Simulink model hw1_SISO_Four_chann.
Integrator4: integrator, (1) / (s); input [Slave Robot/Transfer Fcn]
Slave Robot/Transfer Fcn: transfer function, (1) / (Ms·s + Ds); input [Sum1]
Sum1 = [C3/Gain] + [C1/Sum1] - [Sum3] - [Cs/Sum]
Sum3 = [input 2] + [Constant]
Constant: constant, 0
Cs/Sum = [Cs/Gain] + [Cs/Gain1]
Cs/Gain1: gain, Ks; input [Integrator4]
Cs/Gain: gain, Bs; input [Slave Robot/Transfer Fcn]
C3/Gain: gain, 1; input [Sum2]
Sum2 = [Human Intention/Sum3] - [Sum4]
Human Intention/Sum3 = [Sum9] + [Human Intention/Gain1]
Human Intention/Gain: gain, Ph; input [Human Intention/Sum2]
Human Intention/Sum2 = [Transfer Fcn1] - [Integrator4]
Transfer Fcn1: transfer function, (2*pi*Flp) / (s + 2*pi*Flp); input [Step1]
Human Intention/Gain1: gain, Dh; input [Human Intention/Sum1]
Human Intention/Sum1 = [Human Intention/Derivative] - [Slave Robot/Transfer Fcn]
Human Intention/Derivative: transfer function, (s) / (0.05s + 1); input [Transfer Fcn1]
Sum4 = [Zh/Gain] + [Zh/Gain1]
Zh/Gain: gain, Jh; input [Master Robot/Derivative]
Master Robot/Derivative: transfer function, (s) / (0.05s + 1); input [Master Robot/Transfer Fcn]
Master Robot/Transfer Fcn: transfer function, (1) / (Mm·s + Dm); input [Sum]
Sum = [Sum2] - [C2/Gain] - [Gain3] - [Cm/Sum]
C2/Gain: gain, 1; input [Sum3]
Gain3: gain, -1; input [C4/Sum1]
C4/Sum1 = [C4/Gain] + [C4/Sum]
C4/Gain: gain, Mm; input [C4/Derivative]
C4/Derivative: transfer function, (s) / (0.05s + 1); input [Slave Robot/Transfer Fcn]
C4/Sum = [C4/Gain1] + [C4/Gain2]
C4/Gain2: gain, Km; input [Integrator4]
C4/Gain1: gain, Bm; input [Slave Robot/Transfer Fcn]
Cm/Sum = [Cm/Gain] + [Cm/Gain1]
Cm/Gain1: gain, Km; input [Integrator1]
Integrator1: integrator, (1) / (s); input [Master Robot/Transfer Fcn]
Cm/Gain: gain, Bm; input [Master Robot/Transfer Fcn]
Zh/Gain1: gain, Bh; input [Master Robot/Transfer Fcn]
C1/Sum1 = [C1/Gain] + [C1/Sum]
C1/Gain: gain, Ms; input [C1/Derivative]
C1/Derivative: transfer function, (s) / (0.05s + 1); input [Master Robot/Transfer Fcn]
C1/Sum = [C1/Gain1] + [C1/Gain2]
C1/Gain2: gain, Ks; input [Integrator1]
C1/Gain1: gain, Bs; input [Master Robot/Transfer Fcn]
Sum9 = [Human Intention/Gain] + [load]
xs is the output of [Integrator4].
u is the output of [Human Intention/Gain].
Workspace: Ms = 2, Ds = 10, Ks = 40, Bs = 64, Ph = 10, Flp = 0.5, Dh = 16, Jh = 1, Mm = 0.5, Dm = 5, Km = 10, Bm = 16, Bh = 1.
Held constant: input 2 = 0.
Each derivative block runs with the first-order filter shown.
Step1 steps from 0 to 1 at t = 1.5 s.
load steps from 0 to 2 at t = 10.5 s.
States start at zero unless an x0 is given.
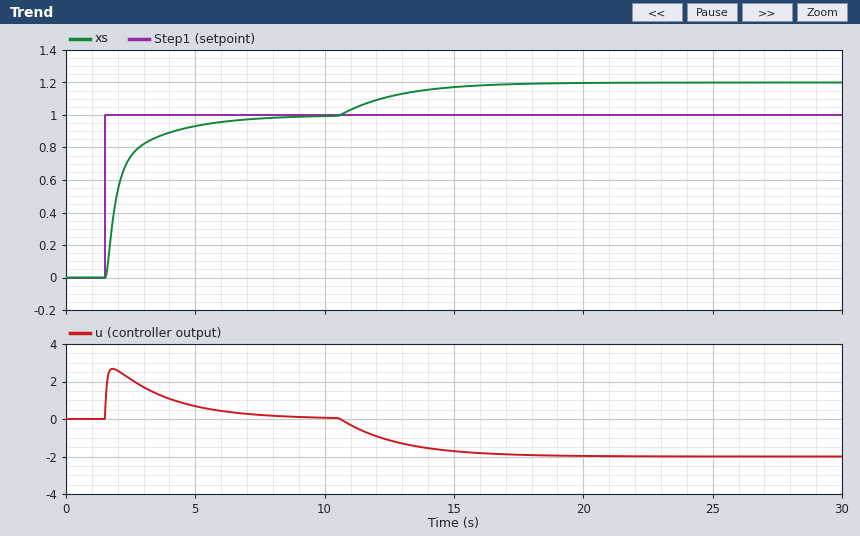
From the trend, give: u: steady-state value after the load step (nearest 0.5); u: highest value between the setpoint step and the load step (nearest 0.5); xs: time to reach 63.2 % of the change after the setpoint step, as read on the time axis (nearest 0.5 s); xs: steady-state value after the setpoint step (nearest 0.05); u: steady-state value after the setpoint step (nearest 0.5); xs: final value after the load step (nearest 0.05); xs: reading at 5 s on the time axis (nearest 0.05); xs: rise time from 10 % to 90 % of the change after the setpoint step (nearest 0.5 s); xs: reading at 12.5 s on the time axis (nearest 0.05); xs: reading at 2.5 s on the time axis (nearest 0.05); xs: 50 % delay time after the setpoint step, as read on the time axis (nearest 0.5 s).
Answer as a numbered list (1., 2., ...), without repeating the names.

1. -2.0
2. 2.5
3. 2.0 s
4. 1.00
5. 0.0
6. 1.20
7. 0.95
8. 2.5 s
9. 1.10
10. 0.75
11. 2.0 s
